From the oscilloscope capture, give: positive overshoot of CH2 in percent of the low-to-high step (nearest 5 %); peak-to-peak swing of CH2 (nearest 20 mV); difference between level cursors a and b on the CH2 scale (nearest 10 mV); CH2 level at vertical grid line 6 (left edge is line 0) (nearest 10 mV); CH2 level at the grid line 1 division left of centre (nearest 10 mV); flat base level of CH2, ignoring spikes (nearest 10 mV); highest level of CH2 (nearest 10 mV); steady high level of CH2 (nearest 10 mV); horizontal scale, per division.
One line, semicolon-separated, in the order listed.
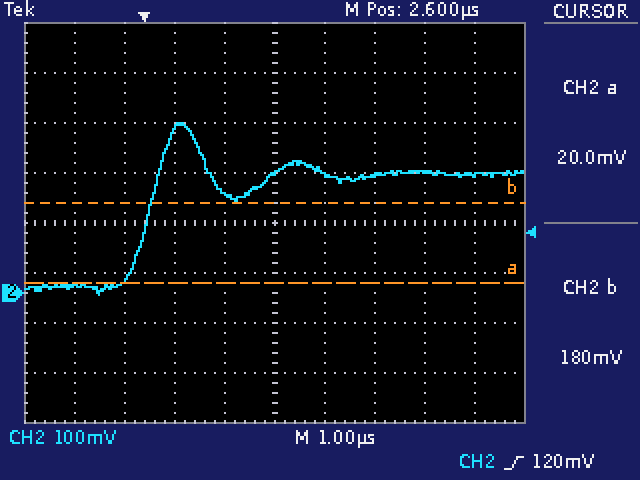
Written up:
45 %; 340 mV; 160 mV; 240 mV; 200 mV; 10 mV; 340 mV; 240 mV; 1 µs
